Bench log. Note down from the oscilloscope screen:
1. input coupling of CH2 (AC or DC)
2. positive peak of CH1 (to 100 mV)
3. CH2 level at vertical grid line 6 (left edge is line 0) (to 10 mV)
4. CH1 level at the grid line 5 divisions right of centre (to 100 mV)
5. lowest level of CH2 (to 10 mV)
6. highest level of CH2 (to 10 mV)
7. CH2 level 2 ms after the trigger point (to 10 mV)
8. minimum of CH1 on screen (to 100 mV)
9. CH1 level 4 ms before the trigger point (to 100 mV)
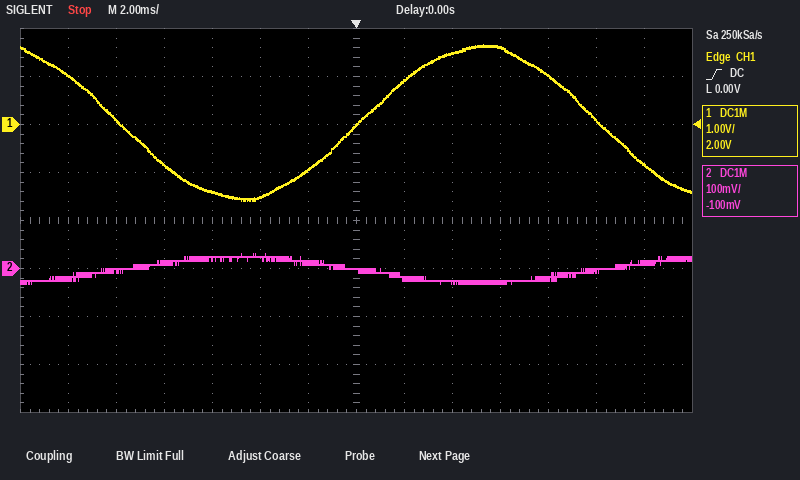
DC
1.7 V
10 mV
100 mV
-30 mV
30 mV
-20 mV
-1.6 V
-1.5 V
